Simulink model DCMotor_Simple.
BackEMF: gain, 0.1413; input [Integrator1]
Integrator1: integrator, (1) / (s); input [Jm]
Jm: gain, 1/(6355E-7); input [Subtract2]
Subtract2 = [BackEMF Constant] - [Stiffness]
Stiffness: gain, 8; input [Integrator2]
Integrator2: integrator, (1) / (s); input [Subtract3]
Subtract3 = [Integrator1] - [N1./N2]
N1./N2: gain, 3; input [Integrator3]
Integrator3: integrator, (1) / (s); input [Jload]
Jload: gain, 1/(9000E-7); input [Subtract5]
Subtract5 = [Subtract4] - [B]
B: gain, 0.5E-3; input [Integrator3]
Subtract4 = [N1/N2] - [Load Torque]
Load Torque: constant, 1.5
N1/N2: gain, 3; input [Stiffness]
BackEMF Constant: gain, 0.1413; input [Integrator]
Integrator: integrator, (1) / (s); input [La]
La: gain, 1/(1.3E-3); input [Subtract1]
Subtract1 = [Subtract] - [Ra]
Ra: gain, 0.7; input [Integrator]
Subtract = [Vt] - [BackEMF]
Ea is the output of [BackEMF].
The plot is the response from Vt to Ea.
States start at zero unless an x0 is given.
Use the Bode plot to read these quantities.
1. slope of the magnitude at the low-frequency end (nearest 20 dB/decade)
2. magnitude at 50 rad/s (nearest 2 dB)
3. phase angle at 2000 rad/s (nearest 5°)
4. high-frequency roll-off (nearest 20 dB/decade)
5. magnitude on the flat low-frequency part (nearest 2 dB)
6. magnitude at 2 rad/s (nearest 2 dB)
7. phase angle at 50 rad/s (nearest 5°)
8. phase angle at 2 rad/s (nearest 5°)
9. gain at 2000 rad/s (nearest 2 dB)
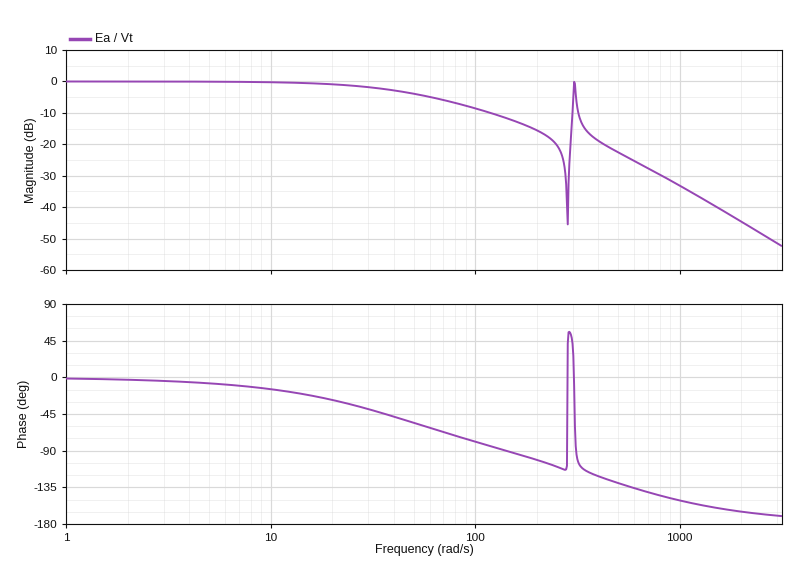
0 dB/decade
-4 dB
-165°
-40 dB/decade
0 dB
0 dB
-55°
-5°
-44 dB
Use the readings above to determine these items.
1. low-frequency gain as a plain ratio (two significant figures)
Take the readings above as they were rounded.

1.0
